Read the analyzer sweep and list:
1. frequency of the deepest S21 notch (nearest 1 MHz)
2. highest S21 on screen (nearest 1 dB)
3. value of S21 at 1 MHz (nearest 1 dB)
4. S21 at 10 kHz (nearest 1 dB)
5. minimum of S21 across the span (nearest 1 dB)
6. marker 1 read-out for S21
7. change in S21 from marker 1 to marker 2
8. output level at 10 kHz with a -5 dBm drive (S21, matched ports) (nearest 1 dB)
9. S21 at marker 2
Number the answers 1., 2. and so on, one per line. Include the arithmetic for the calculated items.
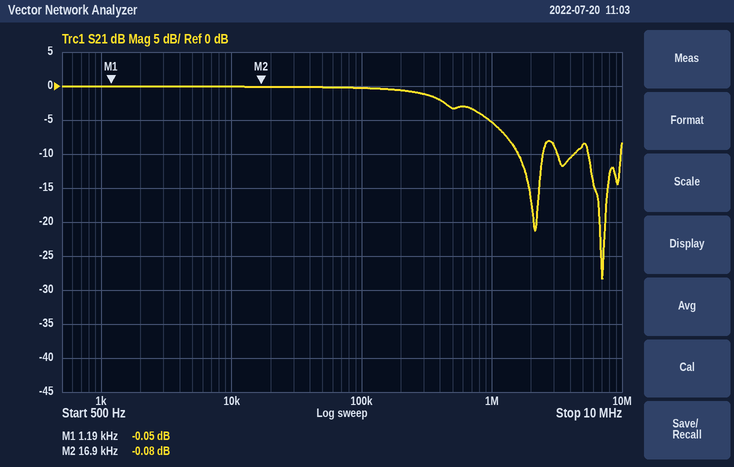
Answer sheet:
1. 7 MHz
2. 0 dB
3. -5 dB
4. 0 dB
5. -28 dB
6. -0.05 dB
7. -0.08 − (-0.05) = -0.03 dB
8. -5 dBm + (0 dB) = -5 dBm
9. -0.08 dB
